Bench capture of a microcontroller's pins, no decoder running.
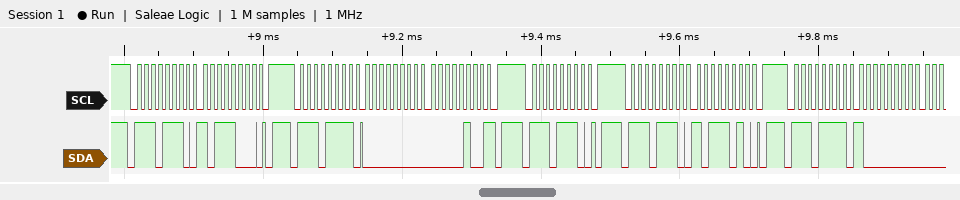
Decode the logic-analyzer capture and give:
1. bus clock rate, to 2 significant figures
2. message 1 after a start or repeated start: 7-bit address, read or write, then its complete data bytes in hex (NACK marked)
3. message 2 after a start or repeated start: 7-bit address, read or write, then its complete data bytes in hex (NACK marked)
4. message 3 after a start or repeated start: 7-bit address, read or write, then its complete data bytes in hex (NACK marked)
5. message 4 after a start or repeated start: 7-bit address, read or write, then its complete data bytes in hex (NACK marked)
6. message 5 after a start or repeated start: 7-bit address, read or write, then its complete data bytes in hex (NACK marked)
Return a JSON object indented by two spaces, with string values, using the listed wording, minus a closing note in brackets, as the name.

{
  "bus clock rate, to 2 significant figures": "100 kHz",
  "message 1 after a start or repeated start: 7-bit address, read or write, then its complete data bytes in hex": "0x77 write: B8",
  "message 2 after a start or repeated start: 7-bit address, read or write, then its complete data bytes in hex": "0x77 read: 00 04 NACK",
  "message 3 after a start or repeated start: 7-bit address, read or write, then its complete data bytes in hex": "0x77 write",
  "message 4 after a start or repeated start: 7-bit address, read or write, then its complete data bytes in hex": "0x77 write: BA",
  "message 5 after a start or repeated start: 7-bit address, read or write, then its complete data bytes in hex": "0x77 read: 80"
}
